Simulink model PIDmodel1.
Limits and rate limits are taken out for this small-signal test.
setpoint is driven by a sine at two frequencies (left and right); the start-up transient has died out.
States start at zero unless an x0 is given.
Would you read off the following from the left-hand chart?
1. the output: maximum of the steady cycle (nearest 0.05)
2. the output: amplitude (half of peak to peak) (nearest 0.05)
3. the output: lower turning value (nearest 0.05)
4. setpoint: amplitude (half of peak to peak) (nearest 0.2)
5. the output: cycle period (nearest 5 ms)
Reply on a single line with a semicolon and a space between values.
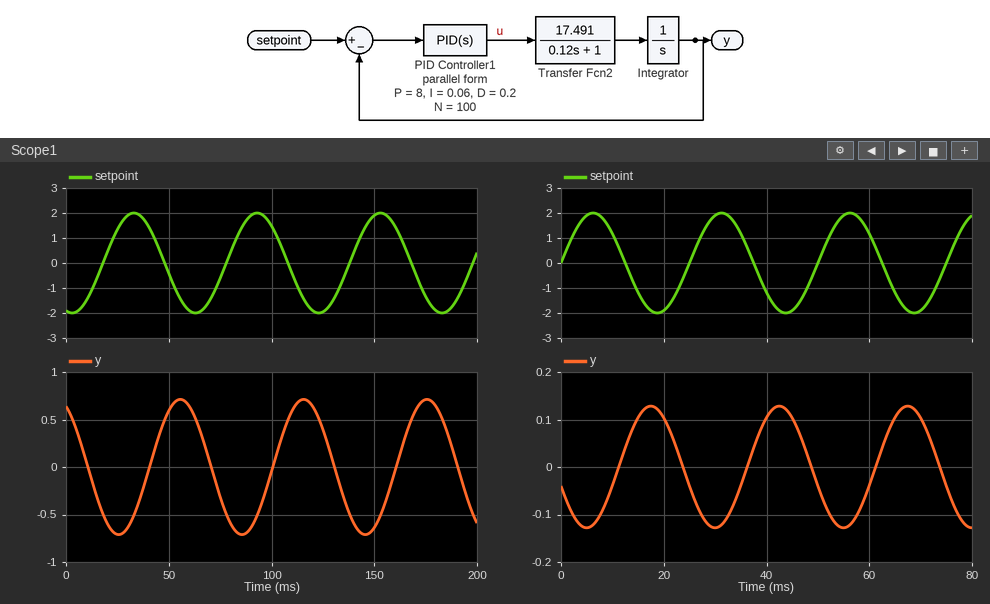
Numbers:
0.70; 0.70; -0.70; 2.0; 60 ms
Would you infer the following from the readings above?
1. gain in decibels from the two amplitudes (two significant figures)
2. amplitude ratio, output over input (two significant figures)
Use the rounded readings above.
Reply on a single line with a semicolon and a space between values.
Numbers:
-9.1 dB; 0.35
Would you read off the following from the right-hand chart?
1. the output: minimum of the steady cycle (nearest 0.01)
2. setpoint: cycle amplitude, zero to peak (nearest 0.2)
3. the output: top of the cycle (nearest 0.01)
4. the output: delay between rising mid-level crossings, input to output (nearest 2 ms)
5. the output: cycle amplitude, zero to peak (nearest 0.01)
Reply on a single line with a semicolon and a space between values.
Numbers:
-0.13; 2.0; 0.13; 12 ms; 0.13
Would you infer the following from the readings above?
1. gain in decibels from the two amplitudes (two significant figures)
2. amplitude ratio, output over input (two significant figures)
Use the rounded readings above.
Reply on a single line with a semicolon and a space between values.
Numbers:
-24 dB; 0.065
